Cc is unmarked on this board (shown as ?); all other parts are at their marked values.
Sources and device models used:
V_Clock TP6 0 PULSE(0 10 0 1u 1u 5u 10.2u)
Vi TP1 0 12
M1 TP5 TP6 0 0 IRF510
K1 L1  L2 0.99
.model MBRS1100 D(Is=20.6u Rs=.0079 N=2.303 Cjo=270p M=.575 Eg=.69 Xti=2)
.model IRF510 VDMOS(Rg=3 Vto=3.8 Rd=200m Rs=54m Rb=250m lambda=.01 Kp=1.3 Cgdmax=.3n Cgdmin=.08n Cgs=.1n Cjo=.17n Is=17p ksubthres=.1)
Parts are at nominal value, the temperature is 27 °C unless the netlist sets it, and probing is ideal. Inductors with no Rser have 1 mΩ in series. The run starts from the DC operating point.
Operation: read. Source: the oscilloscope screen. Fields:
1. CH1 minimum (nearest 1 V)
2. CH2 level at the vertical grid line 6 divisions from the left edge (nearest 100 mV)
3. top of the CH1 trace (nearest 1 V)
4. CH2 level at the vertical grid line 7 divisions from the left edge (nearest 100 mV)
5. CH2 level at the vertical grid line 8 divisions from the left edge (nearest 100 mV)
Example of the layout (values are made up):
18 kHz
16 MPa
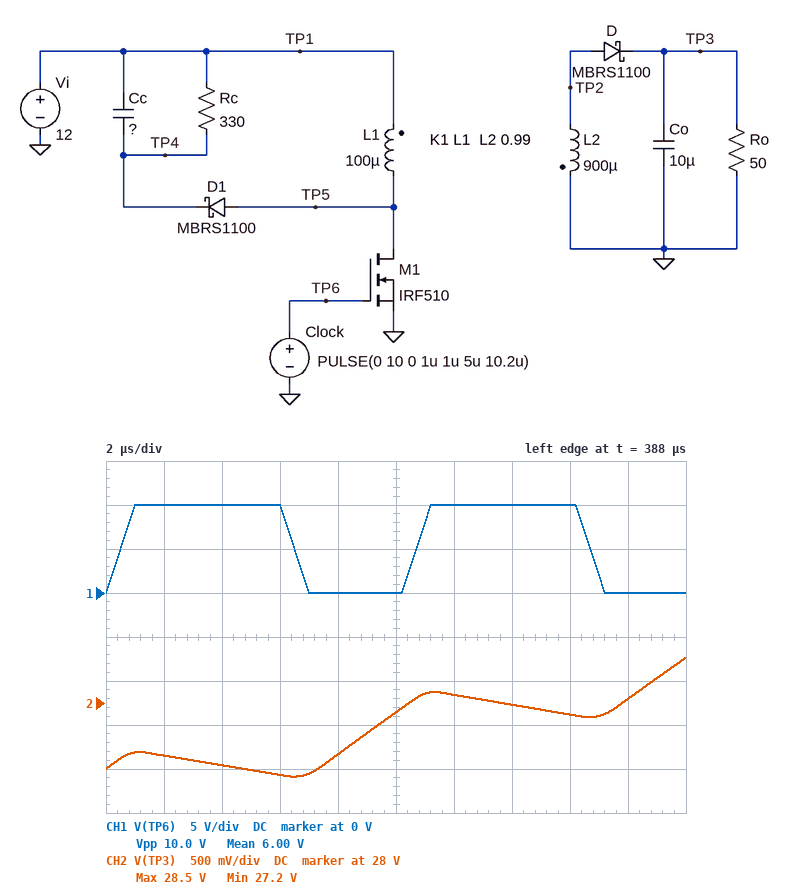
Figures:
0 V
28.1 V
10 V
28.0 V
27.9 V
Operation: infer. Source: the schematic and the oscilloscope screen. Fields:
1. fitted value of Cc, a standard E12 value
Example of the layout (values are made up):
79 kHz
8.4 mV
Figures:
8.2 µF
